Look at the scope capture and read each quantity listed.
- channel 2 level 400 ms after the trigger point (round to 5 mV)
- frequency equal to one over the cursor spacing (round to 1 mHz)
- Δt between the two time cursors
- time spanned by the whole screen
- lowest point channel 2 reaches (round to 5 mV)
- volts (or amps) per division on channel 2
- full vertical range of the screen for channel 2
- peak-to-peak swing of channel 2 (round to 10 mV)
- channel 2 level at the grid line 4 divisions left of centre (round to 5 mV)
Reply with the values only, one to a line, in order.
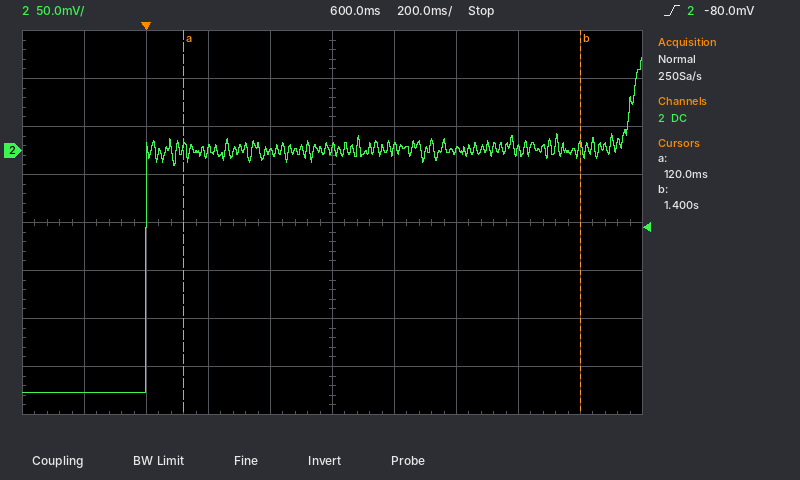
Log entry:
0 mV
781 mHz
1.28 s
2 s
-250 mV
50 mV
400 mV
350 mV
-250 mV
